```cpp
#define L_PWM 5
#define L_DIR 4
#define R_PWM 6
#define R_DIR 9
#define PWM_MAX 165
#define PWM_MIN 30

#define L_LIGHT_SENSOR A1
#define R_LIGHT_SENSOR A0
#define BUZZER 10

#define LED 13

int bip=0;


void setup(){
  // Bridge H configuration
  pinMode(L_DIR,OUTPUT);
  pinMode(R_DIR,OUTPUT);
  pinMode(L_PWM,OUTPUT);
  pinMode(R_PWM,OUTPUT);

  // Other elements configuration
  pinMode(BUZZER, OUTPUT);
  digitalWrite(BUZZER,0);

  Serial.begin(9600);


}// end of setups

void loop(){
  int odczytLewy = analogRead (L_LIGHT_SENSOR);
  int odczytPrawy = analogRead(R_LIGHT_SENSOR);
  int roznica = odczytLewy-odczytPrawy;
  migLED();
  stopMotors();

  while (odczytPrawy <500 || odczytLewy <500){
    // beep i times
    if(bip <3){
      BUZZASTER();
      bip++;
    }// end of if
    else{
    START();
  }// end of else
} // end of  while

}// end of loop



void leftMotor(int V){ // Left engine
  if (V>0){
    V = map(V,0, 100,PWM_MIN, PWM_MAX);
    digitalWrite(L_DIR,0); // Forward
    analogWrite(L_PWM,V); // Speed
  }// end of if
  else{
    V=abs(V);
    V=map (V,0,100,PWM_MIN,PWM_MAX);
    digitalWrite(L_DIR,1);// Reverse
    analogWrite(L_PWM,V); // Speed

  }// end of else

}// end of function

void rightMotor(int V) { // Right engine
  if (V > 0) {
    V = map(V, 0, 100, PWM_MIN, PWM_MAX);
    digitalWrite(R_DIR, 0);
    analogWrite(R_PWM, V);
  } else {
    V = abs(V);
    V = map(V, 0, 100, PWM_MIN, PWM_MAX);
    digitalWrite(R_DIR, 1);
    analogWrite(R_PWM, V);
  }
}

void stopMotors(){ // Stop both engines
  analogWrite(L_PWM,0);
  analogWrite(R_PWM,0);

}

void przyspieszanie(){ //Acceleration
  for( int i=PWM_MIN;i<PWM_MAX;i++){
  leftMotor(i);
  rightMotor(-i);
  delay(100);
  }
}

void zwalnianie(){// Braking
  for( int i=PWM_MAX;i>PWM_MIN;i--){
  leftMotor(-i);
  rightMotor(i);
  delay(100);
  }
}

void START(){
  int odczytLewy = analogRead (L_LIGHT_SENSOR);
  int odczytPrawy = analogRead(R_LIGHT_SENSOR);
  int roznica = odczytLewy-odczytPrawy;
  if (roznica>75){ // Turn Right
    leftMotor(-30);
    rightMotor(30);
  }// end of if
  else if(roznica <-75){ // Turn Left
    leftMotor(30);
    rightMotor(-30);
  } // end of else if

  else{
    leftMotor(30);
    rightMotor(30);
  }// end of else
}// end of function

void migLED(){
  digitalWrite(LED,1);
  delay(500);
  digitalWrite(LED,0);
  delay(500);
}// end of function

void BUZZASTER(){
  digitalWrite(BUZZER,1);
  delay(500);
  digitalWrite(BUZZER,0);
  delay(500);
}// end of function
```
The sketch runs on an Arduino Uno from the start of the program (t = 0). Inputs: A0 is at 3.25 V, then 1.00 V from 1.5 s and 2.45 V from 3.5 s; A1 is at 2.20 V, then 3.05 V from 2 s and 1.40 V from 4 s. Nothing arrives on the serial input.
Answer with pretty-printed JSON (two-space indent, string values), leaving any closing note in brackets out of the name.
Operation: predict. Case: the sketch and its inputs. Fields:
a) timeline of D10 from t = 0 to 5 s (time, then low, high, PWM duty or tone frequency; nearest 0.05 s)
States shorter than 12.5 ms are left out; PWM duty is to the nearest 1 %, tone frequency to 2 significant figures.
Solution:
{
  "timeline of D10 from t = 0 to 5 s": "0 s low; 1 s high; 1.5 s low; 2 s high; 2.5 s low; 3 s high; 3.5 s low"
}
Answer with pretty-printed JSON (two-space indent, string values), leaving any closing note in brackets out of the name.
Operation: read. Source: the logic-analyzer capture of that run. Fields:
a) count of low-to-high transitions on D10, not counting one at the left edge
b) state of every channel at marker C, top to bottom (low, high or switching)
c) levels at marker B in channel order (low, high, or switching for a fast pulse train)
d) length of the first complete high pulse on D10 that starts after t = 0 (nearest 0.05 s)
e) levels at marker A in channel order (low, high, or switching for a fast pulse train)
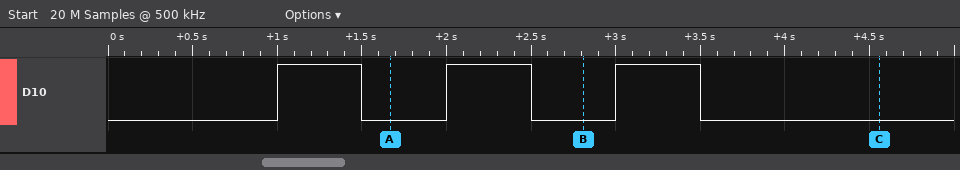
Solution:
{
  "count of low-to-high transitions on D10, not counting one at the left edge": "3",
  "state of every channel at marker C, top to bottom": "D10 low",
  "levels at marker B in channel order": "D10 low",
  "length of the first complete high pulse on D10 that starts after t = 0": "0.50 s",
  "levels at marker A in channel order": "D10 low"
}
